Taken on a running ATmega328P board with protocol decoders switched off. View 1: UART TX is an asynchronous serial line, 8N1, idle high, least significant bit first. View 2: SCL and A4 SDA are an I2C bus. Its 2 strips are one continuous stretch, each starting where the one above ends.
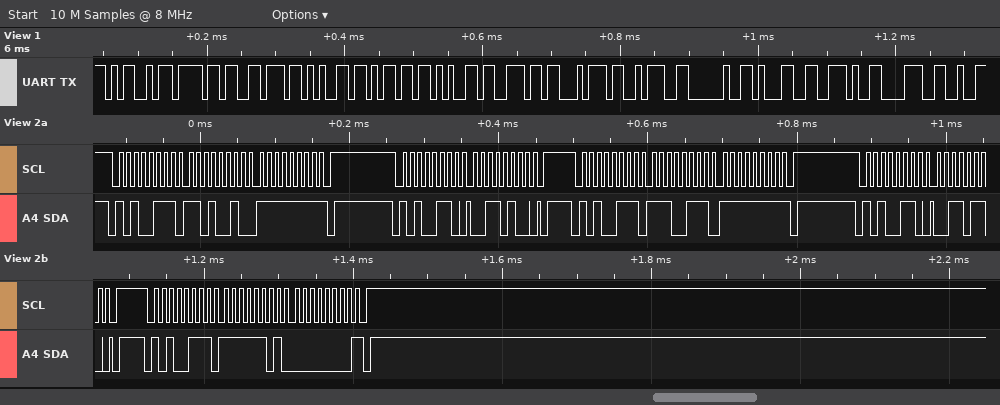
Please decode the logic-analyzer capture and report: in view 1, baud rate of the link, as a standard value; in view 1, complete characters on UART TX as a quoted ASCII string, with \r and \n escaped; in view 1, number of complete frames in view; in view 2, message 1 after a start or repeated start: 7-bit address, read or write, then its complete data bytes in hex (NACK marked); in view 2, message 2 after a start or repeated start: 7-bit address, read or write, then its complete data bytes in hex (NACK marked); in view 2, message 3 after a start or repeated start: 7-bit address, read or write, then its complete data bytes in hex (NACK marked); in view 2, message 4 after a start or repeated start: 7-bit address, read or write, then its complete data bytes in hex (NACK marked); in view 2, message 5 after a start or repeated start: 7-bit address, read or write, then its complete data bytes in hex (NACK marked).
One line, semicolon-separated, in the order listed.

115200 baud; "Movement: 1.8"; 13; 0x53 read: D2 FF NACK; 0x53 write: 34; 0x53 read: E7 FF NACK; 0x53 write: 36; 0x53 read: FD 00 NACK
